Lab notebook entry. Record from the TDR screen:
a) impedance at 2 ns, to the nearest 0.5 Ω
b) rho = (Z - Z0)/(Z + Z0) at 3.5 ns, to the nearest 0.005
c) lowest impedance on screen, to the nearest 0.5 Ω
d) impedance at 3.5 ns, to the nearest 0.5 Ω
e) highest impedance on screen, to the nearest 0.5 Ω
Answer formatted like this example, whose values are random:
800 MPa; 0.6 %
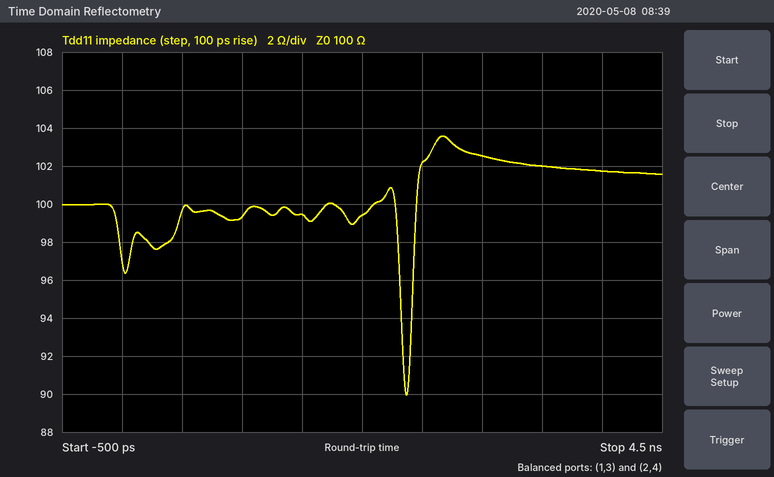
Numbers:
99.5 Ω; +0.010; 90.0 Ω; 102.0 Ω; 103.5 Ω
